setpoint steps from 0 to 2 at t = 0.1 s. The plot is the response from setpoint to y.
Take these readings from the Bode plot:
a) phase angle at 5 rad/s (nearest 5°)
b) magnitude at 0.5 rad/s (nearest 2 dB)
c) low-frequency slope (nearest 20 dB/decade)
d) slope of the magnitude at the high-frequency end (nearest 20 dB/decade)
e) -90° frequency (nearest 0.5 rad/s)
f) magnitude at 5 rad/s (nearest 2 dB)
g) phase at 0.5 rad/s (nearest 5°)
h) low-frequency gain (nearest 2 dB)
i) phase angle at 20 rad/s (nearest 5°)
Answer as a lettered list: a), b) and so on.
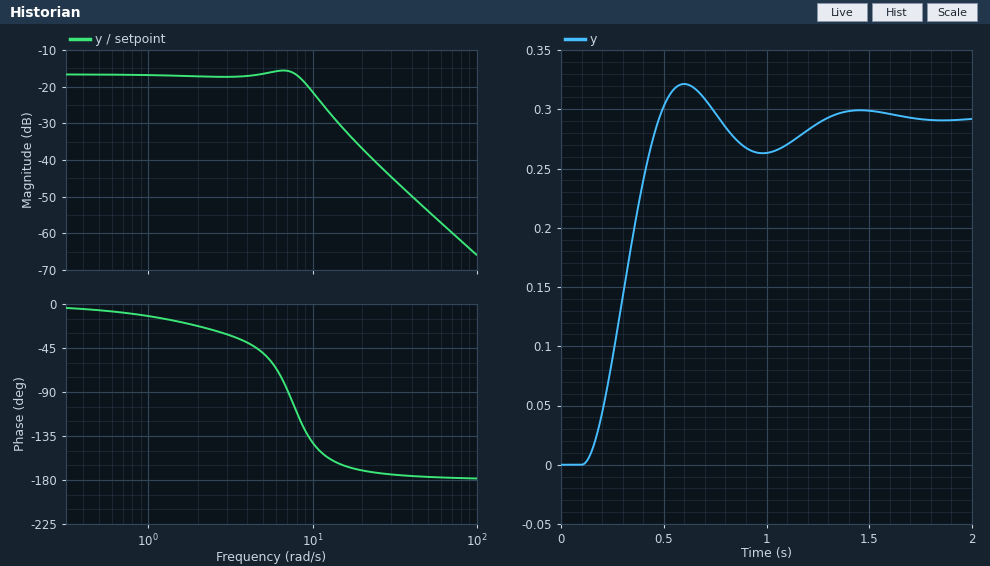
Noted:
a) -50°
b) -16 dB
c) 0 dB/decade
d) -40 dB/decade
e) 7.0 rad/s
f) -16 dB
g) -5°
h) -16 dB
i) -170°
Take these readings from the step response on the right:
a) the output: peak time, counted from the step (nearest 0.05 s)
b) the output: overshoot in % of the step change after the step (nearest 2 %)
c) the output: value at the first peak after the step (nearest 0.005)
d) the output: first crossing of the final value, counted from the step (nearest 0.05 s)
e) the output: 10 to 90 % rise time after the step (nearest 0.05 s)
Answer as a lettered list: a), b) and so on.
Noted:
a) 0.50 s
b) 10 %
c) 0.320
d) 0.40 s
e) 0.25 s
